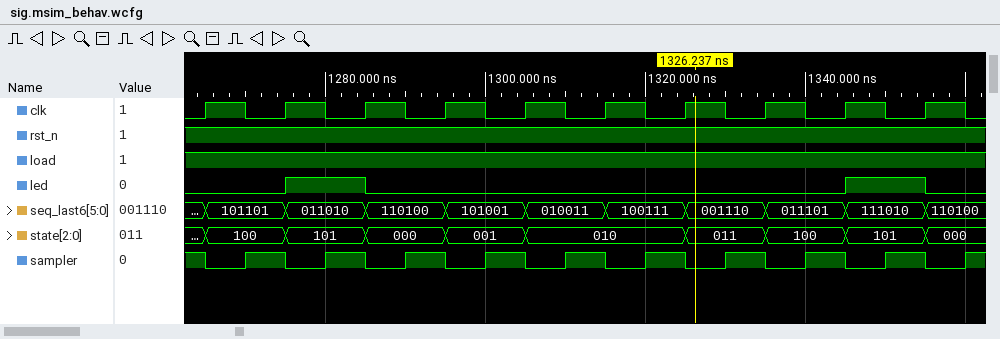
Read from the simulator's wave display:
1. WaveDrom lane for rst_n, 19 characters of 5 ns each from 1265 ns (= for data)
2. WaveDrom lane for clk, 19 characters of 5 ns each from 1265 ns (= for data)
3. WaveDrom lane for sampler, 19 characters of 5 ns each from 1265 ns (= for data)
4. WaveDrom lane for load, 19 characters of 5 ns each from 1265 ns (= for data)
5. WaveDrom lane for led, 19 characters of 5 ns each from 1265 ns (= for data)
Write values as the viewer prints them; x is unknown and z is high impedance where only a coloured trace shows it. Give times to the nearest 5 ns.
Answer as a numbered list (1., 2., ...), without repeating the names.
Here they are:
1. {name: 'rst_n', wave: '1..................'}
2. {name: 'clk', wave: '1010101010101010101'}
3. {name: 'sampler', wave: '0101010101010101010'}
4. {name: 'load', wave: '1..................'}
5. {name: 'led', wave: '0.1.0...........1.0'}
